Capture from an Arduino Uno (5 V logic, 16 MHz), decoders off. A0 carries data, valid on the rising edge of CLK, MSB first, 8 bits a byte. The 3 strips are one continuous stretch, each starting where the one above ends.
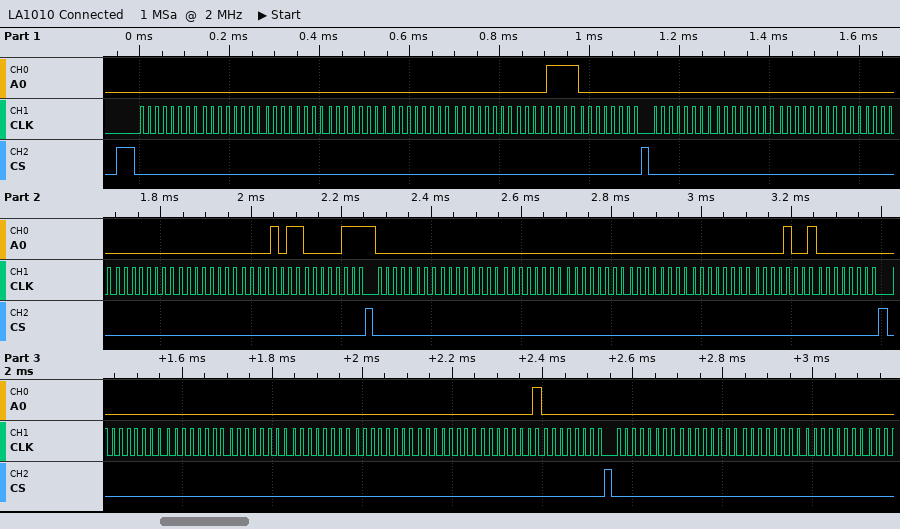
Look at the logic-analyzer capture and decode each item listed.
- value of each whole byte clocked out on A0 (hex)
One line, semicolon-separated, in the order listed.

00 00 00 00 00 00 0F 00 00 00 00 00 00 00 0B 07 00 00 00 00 00 00 09 00 00 00 00 00 00 00 01 00 00 00 00 00
